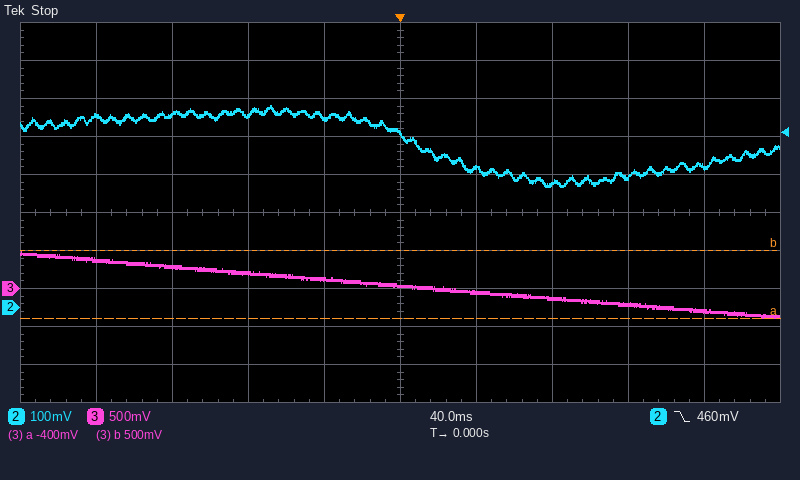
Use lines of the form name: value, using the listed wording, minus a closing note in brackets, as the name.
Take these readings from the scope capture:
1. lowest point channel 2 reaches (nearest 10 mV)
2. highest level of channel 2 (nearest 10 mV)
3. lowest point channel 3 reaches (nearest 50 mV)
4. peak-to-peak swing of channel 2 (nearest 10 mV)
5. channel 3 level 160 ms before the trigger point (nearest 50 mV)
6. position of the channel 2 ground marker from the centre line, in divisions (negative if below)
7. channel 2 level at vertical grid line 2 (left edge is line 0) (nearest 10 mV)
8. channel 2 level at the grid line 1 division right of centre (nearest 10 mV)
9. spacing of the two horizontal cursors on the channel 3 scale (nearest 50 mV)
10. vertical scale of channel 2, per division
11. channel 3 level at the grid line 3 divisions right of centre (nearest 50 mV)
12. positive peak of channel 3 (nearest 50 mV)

lowest point channel 2 reaches: 320 mV
highest level of channel 2: 530 mV
lowest point channel 3 reaches: -400 mV
peak-to-peak swing of channel 2: 210 mV
channel 3 level 160 ms before the trigger point: 400 mV
position of the channel 2 ground marker from the centre line, in divisions: -2.5 div
channel 2 level at vertical grid line 2 (left edge is line 0): 510 mV
channel 2 level at the grid line 1 division right of centre: 370 mV
spacing of the two horizontal cursors on the channel 3 scale: 900 mV
vertical scale of channel 2, per division: 100 mV
channel 3 level at the grid line 3 divisions right of centre: -200 mV
positive peak of channel 3: 500 mV
